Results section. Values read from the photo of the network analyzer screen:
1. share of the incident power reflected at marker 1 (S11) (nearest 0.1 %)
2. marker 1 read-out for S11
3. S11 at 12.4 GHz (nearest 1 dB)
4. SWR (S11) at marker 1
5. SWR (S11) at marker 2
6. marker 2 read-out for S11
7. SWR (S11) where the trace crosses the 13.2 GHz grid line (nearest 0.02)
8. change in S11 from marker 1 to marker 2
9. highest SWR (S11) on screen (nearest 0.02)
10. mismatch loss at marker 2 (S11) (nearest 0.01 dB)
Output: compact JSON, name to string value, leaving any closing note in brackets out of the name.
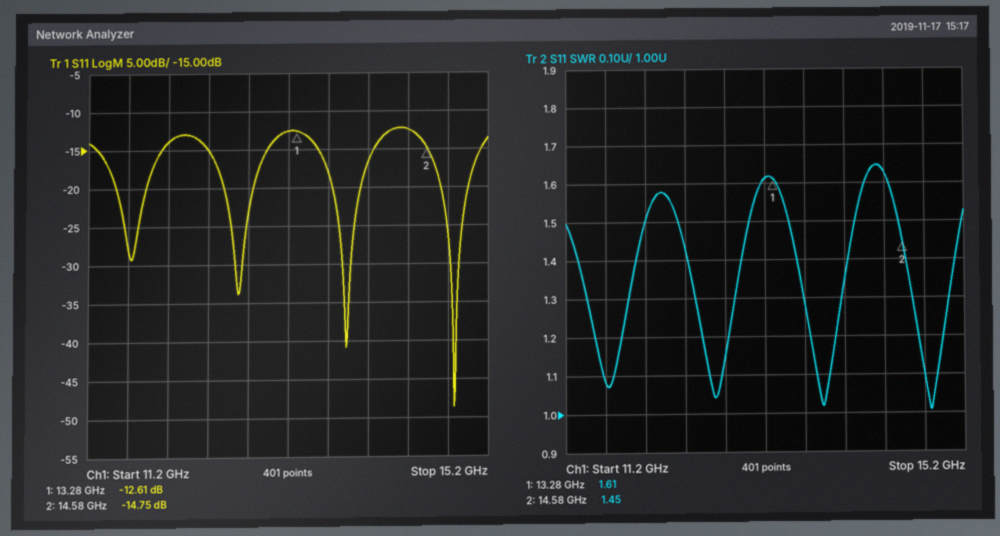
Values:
{"share of the incident power reflected at marker 1 (S11)": "5.5 %", "marker 1 read-out for S11": "-12.61 dB", "S11 at 12.4 GHz": "-15 dB", "SWR (S11) at marker 1": "1.61", "SWR (S11) at marker 2": "1.45", "marker 2 read-out for S11": "-14.75 dB", "SWR (S11) where the trace crosses the 13.2 GHz grid line": "1.62", "change in S11 from marker 1 to marker 2": "-2.14 dB", "highest SWR (S11) on screen": "1.64", "mismatch loss at marker 2 (S11)": "0.15 dB"}
